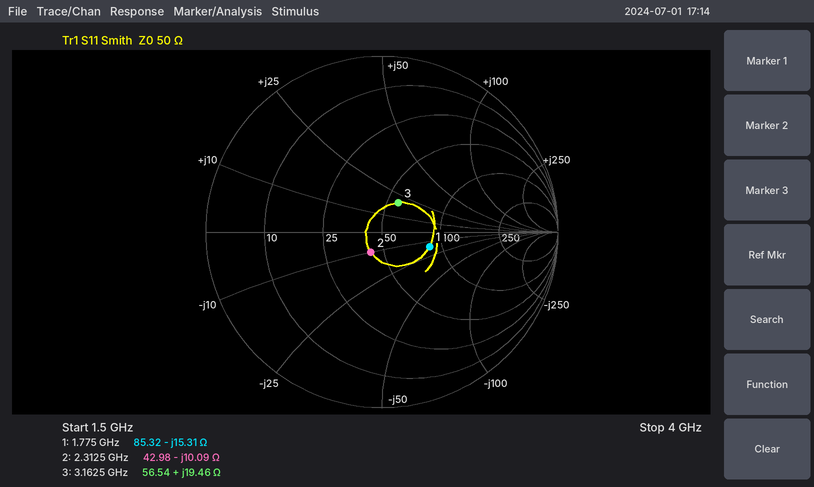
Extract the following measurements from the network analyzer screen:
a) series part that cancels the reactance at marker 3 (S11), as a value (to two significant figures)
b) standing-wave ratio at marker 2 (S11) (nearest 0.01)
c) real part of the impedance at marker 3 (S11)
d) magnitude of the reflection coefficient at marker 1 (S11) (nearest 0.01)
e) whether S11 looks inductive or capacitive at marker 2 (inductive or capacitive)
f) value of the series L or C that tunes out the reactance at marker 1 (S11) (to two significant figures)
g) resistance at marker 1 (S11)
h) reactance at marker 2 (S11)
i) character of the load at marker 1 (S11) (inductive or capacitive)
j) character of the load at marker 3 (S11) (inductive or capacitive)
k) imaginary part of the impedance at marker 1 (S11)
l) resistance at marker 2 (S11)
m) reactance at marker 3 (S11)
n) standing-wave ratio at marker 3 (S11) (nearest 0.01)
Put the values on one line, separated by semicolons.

2.6 pF; 1.30; 56.54 Ω; 0.28; capacitive; 1.4 nH; 85.32 Ω; -10.09 Ω; capacitive; inductive; -15.31 Ω; 42.98 Ω; +19.46 Ω; 1.47
